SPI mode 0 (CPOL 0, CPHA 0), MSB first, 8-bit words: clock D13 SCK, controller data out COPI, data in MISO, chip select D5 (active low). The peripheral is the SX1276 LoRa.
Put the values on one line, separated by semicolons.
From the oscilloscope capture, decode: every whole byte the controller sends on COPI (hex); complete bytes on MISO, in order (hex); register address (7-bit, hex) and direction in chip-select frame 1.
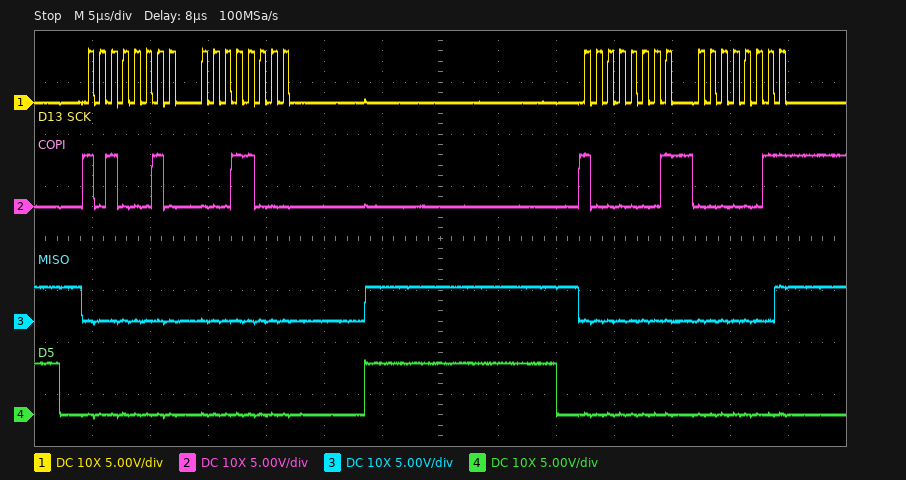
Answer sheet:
A2 18 81 03; 00 00 00 01; 0x22 write
